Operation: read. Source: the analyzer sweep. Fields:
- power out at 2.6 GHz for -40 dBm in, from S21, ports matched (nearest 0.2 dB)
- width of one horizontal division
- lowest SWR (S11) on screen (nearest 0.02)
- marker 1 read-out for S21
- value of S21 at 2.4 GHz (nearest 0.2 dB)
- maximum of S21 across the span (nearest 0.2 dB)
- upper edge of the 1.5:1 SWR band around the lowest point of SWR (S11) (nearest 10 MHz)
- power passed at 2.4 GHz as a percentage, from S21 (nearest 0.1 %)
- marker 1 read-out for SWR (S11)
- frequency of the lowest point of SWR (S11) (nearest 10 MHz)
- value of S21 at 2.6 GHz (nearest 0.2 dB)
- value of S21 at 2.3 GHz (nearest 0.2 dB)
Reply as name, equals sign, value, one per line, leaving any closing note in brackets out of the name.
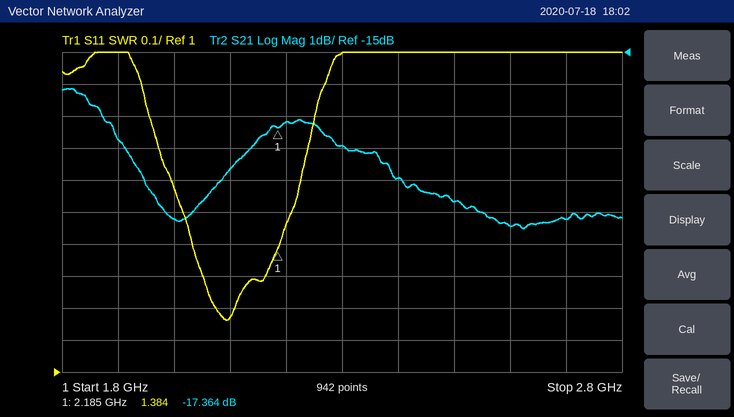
power out at 2.6 GHz for -40 dBm in, from S21, ports matched = -60.4 dBm
width of one horizontal division = 100 MHz
lowest SWR (S11) on screen = 1.16
marker 1 read-out for S21 = -17.364 dB
value of S21 at 2.4 GHz = -19.0 dB
maximum of S21 across the span = -16.2 dB
upper edge of the 1.5:1 SWR band around the lowest point of SWR (S11) = 2.21 GHz
power passed at 2.4 GHz as a percentage, from S21 = 1.3 %
marker 1 read-out for SWR = 1.384
frequency of the lowest point of SWR (S11) = 2.09 GHz
value of S21 at 2.6 GHz = -20.4 dB
value of S21 at 2.3 GHz = -18.0 dB
